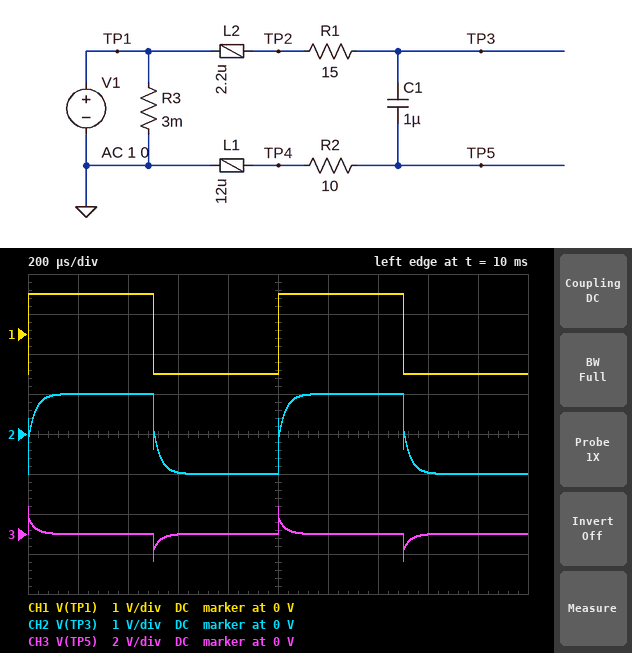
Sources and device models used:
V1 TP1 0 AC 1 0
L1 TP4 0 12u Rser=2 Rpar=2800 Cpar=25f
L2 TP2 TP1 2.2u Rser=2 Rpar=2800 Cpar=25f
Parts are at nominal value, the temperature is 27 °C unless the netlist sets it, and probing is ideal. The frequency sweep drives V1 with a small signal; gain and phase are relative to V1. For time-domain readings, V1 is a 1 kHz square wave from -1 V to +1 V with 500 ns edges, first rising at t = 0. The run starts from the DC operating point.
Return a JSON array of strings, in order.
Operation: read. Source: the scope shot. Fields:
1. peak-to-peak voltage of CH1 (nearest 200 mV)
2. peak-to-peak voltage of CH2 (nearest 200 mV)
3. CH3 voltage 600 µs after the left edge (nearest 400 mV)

["2.0 V", "2.0 V", "0 V"]
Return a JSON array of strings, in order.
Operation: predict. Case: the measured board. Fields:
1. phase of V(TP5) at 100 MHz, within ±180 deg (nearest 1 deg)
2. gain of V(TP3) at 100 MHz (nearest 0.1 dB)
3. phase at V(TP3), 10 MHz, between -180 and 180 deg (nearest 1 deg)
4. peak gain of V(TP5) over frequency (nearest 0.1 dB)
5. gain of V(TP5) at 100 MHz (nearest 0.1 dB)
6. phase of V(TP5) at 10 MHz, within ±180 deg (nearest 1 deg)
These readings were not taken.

["-14 deg", "-2.8 dB", "-1 deg", "-1.5 dB", "-2.8 dB", "-1 deg"]
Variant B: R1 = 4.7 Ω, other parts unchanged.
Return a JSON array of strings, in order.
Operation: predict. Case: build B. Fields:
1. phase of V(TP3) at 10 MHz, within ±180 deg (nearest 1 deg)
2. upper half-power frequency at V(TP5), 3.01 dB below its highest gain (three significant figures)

["-2 deg", "213 MHz"]
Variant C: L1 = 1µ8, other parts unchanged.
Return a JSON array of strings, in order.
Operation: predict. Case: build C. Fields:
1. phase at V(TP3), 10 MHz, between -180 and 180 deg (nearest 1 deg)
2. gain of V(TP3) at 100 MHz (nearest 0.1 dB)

["1 deg", "-6.8 dB"]
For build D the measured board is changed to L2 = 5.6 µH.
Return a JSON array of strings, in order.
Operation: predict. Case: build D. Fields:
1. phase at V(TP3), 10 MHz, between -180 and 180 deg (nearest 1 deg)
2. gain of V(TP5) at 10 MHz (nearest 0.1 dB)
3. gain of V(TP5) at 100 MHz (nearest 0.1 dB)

["-2 deg", "-3.4 dB", "-5.2 dB"]
